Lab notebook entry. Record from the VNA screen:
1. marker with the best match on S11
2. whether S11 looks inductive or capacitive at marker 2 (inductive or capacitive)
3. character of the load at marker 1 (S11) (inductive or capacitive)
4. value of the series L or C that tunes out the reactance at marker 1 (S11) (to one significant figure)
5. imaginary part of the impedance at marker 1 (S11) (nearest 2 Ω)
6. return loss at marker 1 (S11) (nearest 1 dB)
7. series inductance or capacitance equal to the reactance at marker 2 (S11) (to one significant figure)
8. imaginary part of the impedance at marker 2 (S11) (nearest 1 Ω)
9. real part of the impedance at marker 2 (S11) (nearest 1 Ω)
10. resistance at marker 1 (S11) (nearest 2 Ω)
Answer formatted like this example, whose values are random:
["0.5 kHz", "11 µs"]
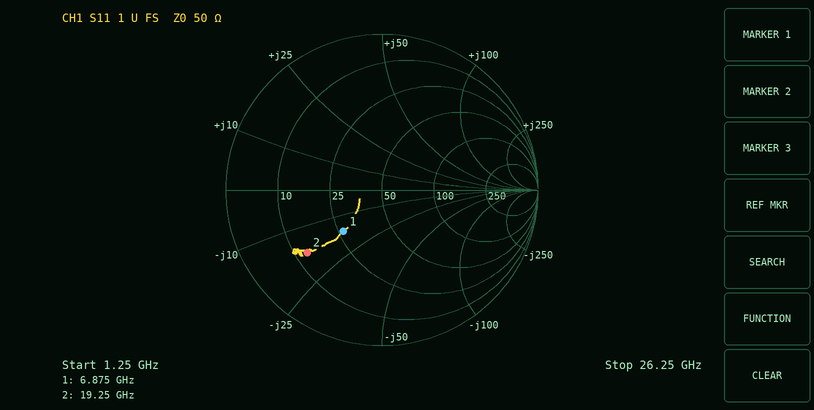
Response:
["marker 1", "capacitive", "capacitive", "400 pH", "-16 Ω", "9 dB", "500 fF", "-17 Ω", "13 Ω", "26 Ω"]
